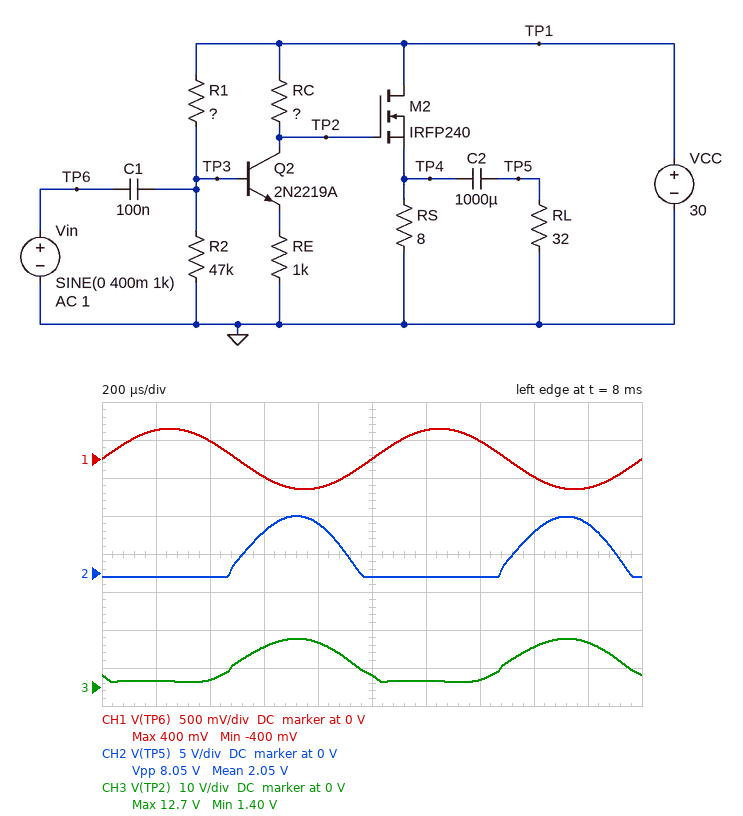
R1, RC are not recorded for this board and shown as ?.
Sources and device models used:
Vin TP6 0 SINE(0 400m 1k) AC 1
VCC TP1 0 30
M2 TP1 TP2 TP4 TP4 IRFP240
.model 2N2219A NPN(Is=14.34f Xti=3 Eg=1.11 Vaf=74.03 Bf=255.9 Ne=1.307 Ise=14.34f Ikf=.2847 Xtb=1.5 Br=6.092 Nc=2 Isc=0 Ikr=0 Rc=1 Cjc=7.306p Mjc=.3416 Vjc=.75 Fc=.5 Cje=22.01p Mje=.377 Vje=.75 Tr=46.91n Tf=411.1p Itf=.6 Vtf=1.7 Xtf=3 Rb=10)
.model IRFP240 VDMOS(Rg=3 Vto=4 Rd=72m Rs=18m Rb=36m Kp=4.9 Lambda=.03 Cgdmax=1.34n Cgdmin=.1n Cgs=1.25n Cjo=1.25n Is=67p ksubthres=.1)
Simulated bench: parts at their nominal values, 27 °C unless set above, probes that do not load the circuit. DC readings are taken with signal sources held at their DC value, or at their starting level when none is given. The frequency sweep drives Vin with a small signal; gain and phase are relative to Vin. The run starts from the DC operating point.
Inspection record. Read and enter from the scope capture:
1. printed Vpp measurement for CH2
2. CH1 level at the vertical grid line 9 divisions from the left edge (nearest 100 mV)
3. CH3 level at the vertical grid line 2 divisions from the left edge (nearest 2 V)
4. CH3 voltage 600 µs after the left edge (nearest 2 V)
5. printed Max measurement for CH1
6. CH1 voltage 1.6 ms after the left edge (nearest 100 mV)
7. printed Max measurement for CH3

8.05 V
-400 mV
2 V
10 V
400 mV
-200 mV
12.7 V
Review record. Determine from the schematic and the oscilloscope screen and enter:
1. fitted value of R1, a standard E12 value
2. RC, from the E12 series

330 kΩ
22 kΩ
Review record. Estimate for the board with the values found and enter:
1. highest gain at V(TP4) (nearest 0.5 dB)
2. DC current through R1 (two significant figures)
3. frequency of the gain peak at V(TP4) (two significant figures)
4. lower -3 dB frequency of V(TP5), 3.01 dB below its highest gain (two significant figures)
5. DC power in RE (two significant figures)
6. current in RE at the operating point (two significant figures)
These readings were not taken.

-13.0 dB
85 µA
56 MHz
19 MHz
1.8 mW
1.3 mA
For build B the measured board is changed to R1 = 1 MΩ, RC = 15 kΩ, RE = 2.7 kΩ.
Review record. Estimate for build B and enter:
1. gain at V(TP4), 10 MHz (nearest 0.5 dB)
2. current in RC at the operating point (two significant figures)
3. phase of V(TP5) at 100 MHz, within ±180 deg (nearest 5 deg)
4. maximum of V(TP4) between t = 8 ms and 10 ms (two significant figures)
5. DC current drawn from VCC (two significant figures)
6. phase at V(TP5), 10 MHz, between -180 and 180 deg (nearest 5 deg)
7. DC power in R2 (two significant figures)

-33.5 dB
250 µA
-10 deg
23 V
2.7 A
55 deg
35 µW
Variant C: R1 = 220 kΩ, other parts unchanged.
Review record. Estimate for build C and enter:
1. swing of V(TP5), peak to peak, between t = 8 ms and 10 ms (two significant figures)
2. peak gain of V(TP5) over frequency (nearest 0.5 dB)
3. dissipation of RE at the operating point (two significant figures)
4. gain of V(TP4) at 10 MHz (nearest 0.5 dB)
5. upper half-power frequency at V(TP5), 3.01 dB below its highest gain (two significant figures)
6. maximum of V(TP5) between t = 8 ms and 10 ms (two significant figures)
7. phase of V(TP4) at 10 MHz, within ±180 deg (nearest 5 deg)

4.6 V
-12.0 dB
1.9 mW
-16.5 dB
150 MHz
4.3 V
50 deg
